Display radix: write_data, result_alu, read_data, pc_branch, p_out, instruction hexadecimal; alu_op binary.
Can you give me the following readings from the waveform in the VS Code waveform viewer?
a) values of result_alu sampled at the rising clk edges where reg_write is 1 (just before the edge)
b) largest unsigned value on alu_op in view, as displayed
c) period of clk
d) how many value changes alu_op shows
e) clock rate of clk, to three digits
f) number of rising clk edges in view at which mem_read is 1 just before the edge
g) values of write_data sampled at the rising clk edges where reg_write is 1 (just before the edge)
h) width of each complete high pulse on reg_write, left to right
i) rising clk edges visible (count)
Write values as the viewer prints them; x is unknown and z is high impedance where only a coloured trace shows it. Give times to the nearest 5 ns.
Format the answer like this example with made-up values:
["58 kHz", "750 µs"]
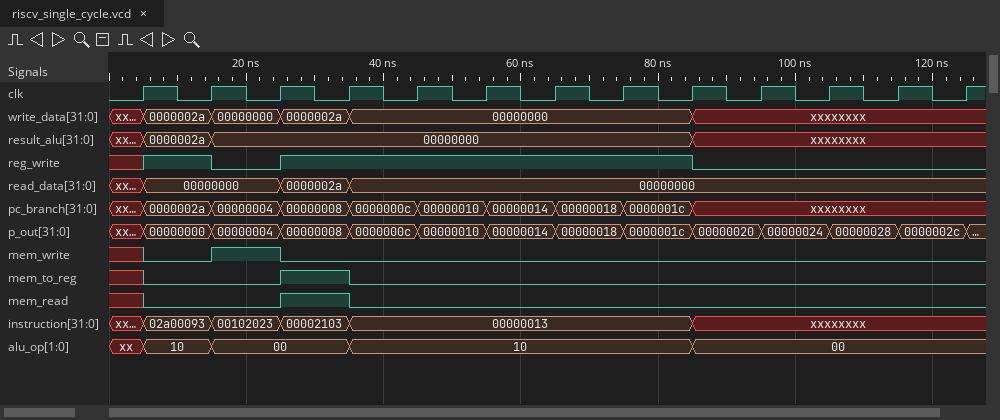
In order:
["0000002a, 00000000, 00000000, 00000000, 00000000, 00000000, 00000000", "10", "10 ns", "4", "100 MHz", "1", "0000002a, 0000002a, 00000000, 00000000, 00000000, 00000000, 00000000", "60 ns", "13"]
